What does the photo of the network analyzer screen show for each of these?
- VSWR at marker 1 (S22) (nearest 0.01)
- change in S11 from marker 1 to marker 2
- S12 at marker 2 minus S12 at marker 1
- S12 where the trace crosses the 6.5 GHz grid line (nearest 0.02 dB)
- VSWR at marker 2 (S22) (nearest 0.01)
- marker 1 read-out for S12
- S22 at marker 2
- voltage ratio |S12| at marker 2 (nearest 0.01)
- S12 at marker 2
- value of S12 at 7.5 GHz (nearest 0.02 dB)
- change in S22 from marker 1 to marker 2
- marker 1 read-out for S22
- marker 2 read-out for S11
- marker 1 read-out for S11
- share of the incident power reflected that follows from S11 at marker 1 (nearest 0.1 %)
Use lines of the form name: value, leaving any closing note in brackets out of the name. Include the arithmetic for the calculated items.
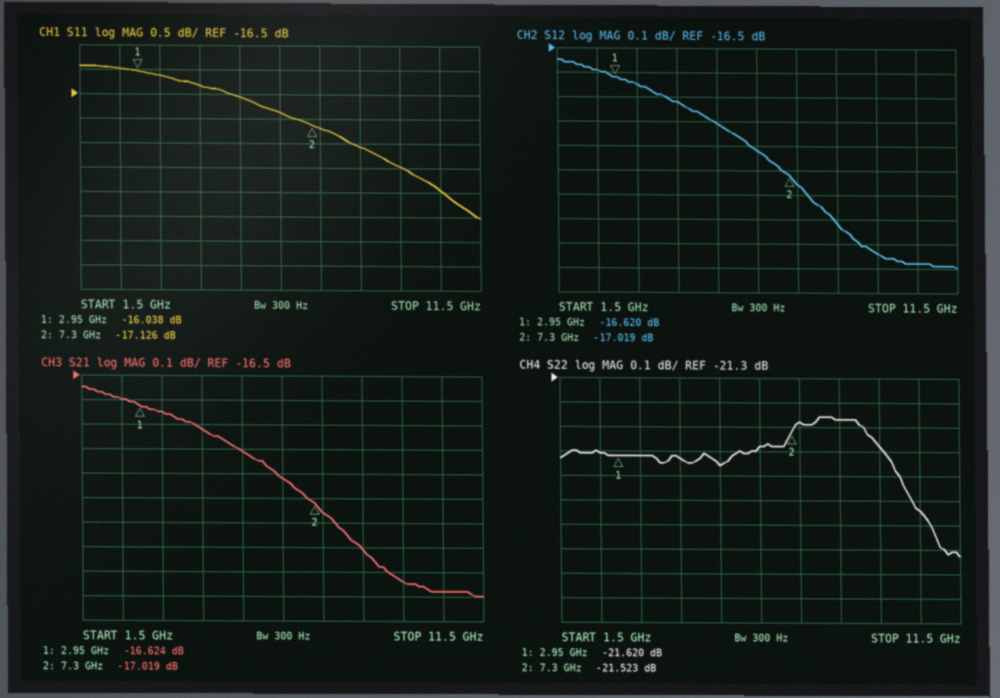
VSWR at marker 1 (S22): (1 + 0.0830)/(1 − 0.0830) ≈ 1.18
change in S11 from marker 1 to marker 2: -17.126 − (-16.038) = -1.088 dB
S12 at marker 2 minus S12 at marker 1: -17.019 − (-16.62) = -0.399 dB
S12 where the trace crosses the 6.5 GHz grid line: -16.92 dB
VSWR at marker 2 (S22): (1 + 0.0839)/(1 − 0.0839) ≈ 1.18
marker 1 read-out for S12: -16.620 dB
S22 at marker 2: -21.523 dB
voltage ratio |S12| at marker 2: 10^(-17.019/20) ≈ 0.14
S12 at marker 2: -17.019 dB
value of S12 at 7.5 GHz: -17.06 dB
change in S22 from marker 1 to marker 2: -21.523 − (-21.62) = 0.097 dB
marker 1 read-out for S22: -21.620 dB
marker 2 read-out for S11: -17.126 dB
marker 1 read-out for S11: -16.038 dB
share of the incident power reflected that follows from S11 at marker 1: 10^(-16.038/10) ≈ 2.5 %
